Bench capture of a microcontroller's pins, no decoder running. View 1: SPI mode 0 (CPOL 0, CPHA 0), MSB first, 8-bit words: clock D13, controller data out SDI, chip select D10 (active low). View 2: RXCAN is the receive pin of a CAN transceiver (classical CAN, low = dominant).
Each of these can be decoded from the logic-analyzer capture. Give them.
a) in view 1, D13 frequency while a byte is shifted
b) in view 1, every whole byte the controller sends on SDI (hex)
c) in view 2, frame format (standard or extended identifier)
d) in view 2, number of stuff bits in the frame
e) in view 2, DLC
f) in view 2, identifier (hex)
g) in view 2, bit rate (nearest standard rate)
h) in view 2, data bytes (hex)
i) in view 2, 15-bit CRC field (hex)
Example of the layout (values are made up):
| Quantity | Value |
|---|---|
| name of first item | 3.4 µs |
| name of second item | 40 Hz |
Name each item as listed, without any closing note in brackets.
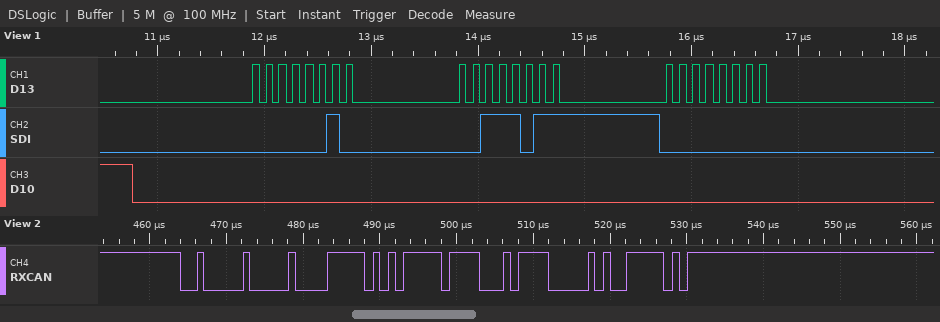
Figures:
| Quantity | Value |
|---|---|
| in view 1, D13 frequency while a byte is shifted | 8 MHz |
| in view 1, every whole byte the controller sends on SDI | 02 3B 00 |
| in view 2, frame format | standard |
| in view 2, number of stuff bits in the frame | 6 |
| in view 2, DLC | 3 |
| in view 2, identifier | 0x200 |
| in view 2, bit rate | 1000 kbit/s |
| in view 2, data bytes | F5 FF 17 |
| in view 2, 15-bit CRC field | 0x409F |
